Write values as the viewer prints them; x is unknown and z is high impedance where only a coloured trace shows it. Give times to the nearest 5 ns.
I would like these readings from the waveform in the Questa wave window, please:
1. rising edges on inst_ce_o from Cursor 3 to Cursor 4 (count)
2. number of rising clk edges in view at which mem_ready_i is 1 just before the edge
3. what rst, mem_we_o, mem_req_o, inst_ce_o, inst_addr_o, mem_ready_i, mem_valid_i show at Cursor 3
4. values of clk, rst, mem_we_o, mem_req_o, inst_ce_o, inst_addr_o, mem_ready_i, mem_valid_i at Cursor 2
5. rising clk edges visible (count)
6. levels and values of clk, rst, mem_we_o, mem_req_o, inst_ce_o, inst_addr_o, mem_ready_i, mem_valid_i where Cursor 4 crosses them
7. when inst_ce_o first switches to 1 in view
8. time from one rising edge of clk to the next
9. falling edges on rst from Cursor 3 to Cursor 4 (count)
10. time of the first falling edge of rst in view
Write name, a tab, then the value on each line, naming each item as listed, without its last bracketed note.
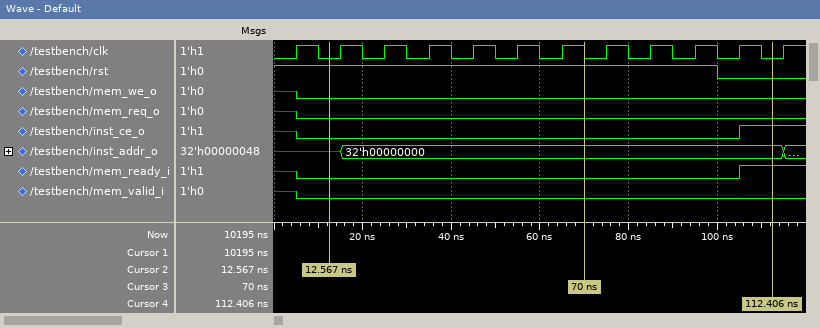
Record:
rising edges on inst_ce_o from Cursor 3 to Cursor 4	1
number of rising clk edges in view at which mem_ready_i is 1 just before the edge	1
what rst, mem_we_o, mem_req_o, inst_ce_o, inst_addr_o, mem_ready_i, mem_valid_i show at Cursor 3	rst=1, mem_we_o=0, mem_req_o=0, inst_ce_o=0, inst_addr_o=32'h00000000, mem_ready_i=0, mem_valid_i=0
values of clk, rst, mem_we_o, mem_req_o, inst_ce_o, inst_addr_o, mem_ready_i, mem_valid_i at Cursor 2	clk=0, rst=1, mem_we_o=0, mem_req_o=0, inst_ce_o=0, inst_addr_o=x, mem_ready_i=0, mem_valid_i=0
rising clk edges visible	12
levels and values of clk, rst, mem_we_o, mem_req_o, inst_ce_o, inst_addr_o, mem_ready_i, mem_valid_i where Cursor 4 crosses them	clk=0, rst=0, mem_we_o=0, mem_req_o=0, inst_ce_o=1, inst_addr_o=32'h00000000, mem_ready_i=1, mem_valid_i=0
when inst_ce_o first switches to 1 in view	105 ns
time from one rising edge of clk to the next	10 ns
falling edges on rst from Cursor 3 to Cursor 4	1
time of the first falling edge of rst in view	100 ns
